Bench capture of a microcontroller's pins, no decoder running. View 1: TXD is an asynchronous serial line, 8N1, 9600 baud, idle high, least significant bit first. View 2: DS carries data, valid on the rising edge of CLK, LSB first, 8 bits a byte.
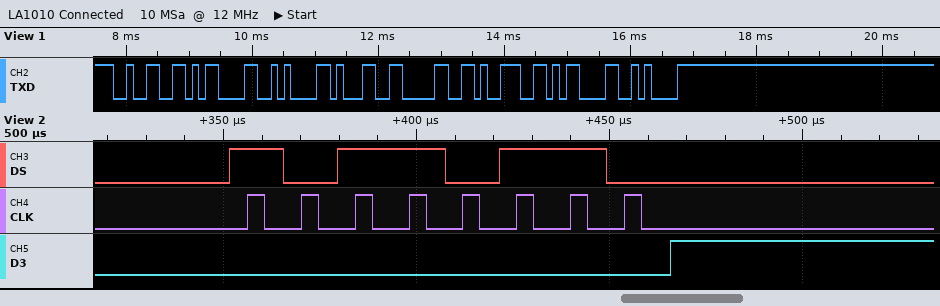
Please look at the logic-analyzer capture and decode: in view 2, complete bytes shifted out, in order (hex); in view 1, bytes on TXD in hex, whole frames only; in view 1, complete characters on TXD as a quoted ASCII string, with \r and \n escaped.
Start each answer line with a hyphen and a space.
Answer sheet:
- 0x6D
- 32 0D 0A 31 30 39 0D 0A
- "2\r\n109\r\n"
